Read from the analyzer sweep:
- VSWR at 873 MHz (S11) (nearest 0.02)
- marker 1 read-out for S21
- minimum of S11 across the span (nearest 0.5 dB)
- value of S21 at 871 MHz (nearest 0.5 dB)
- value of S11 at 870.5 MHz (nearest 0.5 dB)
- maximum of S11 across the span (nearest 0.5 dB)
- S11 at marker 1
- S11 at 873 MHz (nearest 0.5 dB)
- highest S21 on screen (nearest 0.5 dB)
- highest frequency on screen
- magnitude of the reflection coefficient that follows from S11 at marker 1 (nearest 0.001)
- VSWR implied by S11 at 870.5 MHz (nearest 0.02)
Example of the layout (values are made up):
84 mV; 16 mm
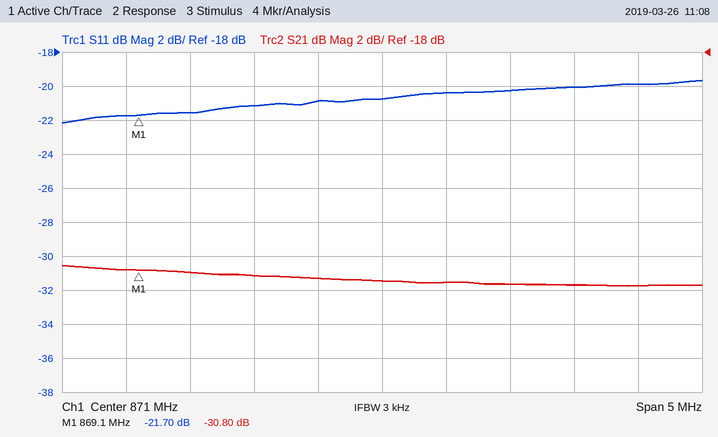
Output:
1.22; -30.80 dB; -22.0 dB; -31.5 dB; -21.0 dB; -19.5 dB; -21.70 dB; -20.0 dB; -30.5 dB; 873.5 MHz; 0.082; 1.20
